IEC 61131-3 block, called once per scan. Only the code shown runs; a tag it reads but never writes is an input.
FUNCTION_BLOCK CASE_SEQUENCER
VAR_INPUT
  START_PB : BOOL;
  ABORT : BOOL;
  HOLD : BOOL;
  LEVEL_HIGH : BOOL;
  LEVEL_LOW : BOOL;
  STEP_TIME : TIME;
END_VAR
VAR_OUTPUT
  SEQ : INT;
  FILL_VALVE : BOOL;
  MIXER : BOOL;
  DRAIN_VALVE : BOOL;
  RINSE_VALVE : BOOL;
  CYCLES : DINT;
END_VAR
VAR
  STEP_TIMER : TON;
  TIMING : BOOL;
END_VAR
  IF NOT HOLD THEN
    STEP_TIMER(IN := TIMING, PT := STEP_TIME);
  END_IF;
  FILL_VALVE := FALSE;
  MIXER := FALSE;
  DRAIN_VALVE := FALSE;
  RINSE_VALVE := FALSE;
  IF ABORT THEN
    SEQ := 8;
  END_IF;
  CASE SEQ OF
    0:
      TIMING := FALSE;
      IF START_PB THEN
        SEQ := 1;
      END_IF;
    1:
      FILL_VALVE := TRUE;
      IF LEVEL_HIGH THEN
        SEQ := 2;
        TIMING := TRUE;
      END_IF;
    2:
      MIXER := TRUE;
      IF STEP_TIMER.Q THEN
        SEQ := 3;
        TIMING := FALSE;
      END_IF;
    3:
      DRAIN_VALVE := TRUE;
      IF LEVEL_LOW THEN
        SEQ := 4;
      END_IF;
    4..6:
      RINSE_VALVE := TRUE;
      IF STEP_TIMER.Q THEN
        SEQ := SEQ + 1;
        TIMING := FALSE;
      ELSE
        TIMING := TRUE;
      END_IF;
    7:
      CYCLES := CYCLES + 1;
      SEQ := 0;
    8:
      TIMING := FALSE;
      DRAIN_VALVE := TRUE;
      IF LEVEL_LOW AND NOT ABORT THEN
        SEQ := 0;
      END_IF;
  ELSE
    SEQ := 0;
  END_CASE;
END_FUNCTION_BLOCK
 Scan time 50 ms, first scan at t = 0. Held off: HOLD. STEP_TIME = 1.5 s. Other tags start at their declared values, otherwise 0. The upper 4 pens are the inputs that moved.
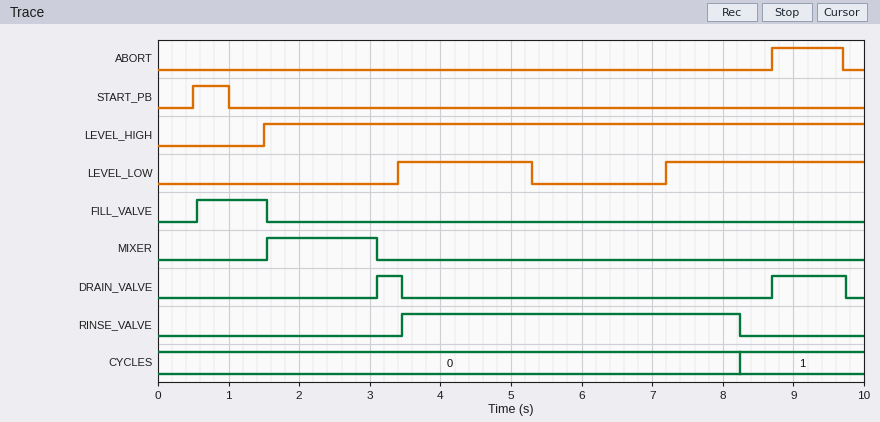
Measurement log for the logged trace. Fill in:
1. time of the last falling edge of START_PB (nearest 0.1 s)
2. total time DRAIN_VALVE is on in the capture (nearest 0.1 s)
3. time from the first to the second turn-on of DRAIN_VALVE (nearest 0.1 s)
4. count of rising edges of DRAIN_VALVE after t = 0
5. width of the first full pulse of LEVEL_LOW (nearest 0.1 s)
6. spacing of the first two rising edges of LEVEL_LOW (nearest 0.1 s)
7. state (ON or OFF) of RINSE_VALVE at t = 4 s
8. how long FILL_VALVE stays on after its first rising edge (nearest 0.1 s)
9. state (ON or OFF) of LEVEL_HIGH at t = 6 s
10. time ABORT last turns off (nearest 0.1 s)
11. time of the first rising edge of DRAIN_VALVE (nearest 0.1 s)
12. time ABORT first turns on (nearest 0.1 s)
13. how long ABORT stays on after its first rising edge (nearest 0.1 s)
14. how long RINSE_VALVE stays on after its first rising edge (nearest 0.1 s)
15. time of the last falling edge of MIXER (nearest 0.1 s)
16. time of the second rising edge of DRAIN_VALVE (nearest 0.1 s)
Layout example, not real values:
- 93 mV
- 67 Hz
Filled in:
- 1.0 s
- 1.4 s
- 5.6 s
- 2
- 1.9 s
- 3.8 s
- ON
- 1.0 s
- ON
- 9.7 s
- 3.1 s
- 8.7 s
- 1.0 s
- 4.8 s
- 3.1 s
- 8.7 s
